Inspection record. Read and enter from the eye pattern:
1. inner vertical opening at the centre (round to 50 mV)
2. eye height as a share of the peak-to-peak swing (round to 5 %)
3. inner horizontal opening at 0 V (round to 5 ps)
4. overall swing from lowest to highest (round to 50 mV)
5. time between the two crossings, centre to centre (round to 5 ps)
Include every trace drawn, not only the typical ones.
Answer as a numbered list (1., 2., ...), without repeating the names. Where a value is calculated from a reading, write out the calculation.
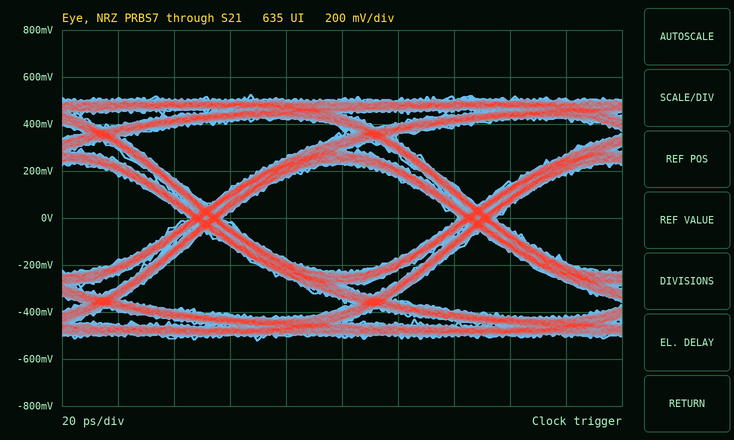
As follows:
1. 450 mV
2. 450 mV / 1.05 V ≈ 42.9 %, so 45 % to the nearest 5 %
3. 85 ps
4. 1.05 V
5. 95 ps
